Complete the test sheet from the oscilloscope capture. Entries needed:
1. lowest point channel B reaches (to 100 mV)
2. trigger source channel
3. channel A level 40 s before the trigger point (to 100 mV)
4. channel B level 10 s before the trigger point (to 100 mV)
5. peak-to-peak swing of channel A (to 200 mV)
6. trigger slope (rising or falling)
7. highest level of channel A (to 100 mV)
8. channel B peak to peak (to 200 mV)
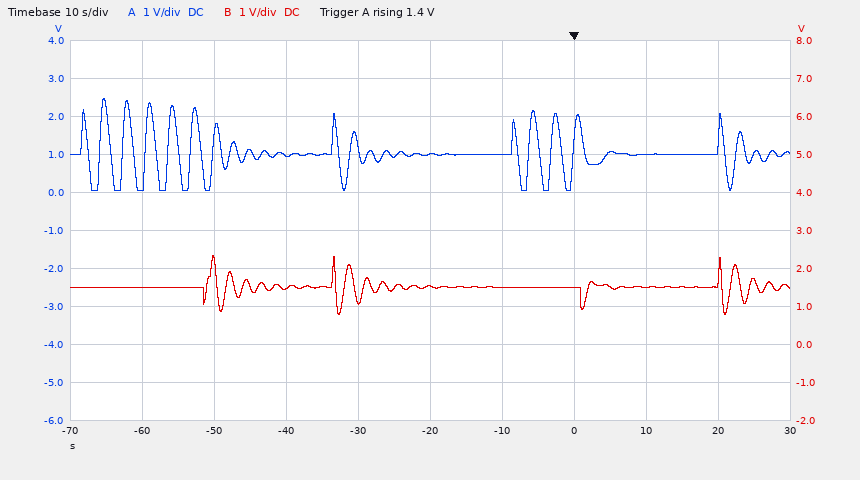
800 mV
channel A
1.0 V
1.5 V
2.4 V
rising
2.5 V
1.6 V
